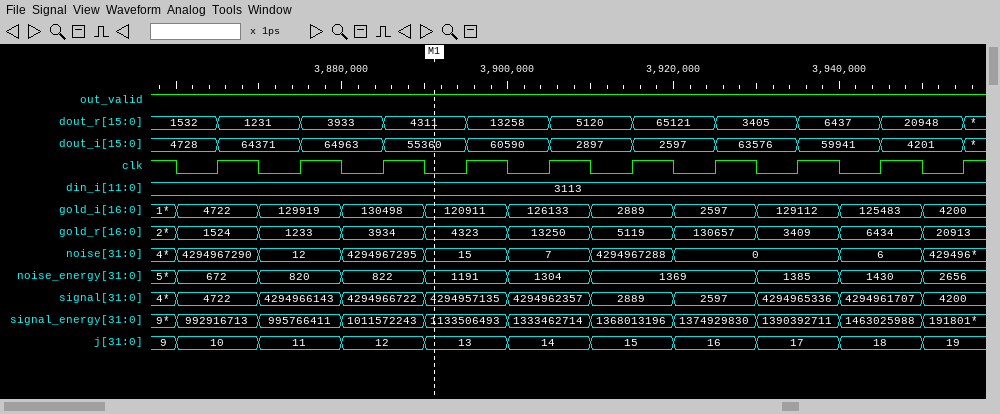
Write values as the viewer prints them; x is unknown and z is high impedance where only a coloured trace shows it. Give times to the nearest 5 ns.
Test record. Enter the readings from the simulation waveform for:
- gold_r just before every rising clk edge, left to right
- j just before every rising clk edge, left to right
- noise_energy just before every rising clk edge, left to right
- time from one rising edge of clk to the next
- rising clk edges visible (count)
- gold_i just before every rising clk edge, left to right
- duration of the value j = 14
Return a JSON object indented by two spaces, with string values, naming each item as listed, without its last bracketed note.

{
  "gold_r just before every rising clk edge, left to right": "1524, 1233, 3934, 4323, 13250, 5119, 130657, 3409, 6434, 20913",
  "j just before every rising clk edge, left to right": "10, 11, 12, 13, 14, 15, 16, 17, 18, 19",
  "noise_energy just before every rising clk edge, left to right": "672, 820, 822, 1191, 1304, 1369, 1369, 1385, 1430, 2656",
  "time from one rising edge of clk to the next": "10 ns",
  "rising clk edges visible": "10",
  "gold_i just before every rising clk edge, left to right": "4722, 129919, 130498, 120911, 126133, 2889, 2597, 129112, 125483, 4200",
  "duration of the value j = 14": "10 ns"
}
